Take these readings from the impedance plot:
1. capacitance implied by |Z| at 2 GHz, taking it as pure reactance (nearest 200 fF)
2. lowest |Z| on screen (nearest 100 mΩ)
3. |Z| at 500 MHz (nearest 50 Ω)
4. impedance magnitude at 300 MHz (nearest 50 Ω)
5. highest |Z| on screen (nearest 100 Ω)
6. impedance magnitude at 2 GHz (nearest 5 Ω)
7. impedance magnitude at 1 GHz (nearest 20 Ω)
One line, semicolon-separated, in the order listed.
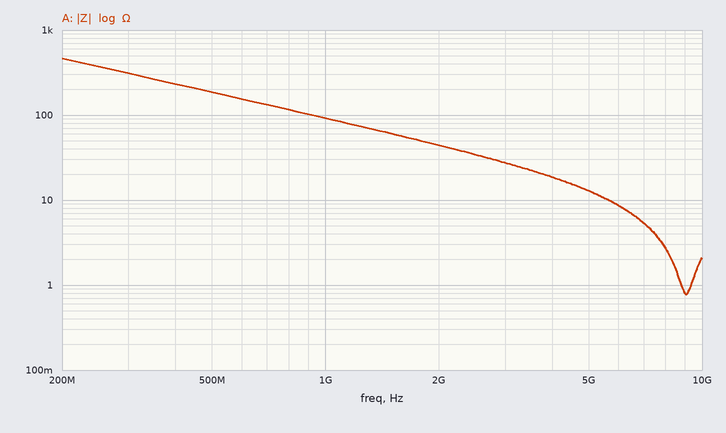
1.8 pF; 800 mΩ; 200 Ω; 300 Ω; 500 Ω; 45 Ω; 100 Ω
